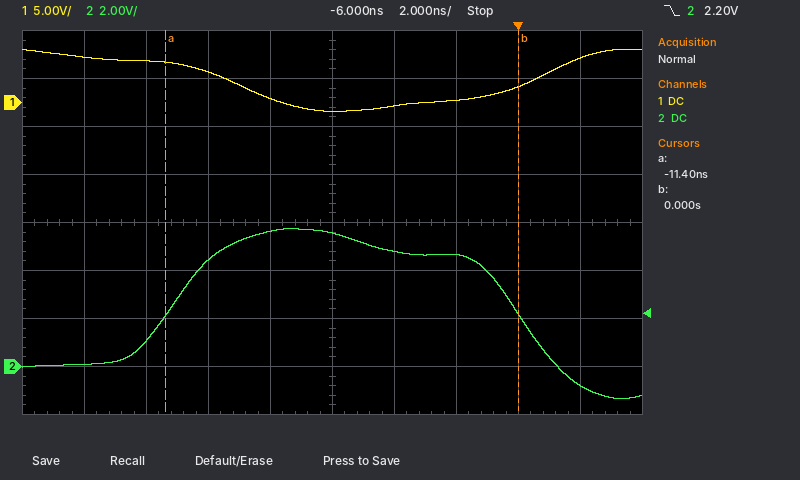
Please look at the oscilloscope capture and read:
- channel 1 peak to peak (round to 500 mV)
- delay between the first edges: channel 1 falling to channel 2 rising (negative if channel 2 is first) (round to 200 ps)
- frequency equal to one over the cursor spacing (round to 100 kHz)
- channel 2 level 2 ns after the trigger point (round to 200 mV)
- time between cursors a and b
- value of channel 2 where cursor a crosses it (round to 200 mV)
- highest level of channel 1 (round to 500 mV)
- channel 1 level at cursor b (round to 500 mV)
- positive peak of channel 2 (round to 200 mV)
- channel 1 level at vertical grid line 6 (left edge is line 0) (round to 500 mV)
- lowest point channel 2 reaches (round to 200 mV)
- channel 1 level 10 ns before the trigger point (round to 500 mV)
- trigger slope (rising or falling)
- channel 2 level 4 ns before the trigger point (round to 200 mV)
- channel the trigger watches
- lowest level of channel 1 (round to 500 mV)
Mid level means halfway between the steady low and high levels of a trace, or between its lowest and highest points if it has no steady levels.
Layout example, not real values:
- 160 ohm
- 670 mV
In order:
- 6.5 V
- -2.0 ns
- 87.7 MHz
- -800 mV
- 11.4 ns
- 2.2 V
- 5.5 V
- 1.5 V
- 5.8 V
- -500 mV
- -1.4 V
- 3.0 V
- falling
- 4.8 V
- channel 2
- -1.0 V
